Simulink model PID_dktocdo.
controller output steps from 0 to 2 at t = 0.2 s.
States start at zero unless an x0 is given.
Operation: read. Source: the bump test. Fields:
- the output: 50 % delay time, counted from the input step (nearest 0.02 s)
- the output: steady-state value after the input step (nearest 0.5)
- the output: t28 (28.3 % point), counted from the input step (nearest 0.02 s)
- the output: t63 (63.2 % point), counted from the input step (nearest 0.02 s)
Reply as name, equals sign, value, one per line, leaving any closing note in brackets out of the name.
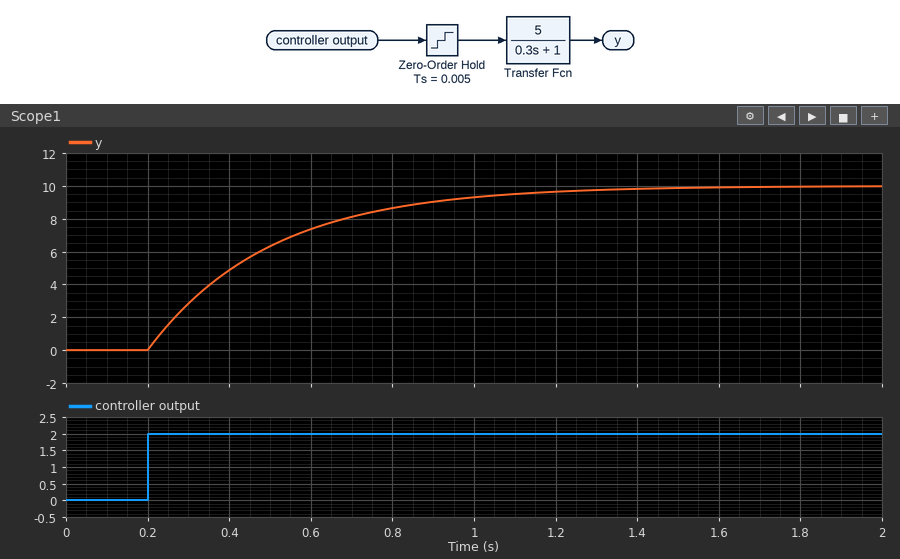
the output: 50 % delay time, counted from the input step = 0.20 s
the output: steady-state value after the input step = 10.0
the output: t28 (28.3 % point), counted from the input step = 0.10 s
the output: t63 (63.2 % point), counted from the input step = 0.30 s
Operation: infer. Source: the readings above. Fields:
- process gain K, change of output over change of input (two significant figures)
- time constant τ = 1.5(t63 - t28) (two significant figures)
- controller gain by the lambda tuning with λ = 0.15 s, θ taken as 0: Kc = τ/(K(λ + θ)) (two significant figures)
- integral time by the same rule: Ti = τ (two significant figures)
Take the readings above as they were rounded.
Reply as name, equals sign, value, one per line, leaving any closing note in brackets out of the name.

process gain K, change of output over change of input = 5.0
time constant τ = 1.5(t63 - t28) = 0.30 s
controller gain by the lambda tuning with λ = 0.15 s, θ taken as 0: Kc = τ/(K(λ + θ)) = 0.40
integral time by the same rule: Ti = τ = 0.30 s
